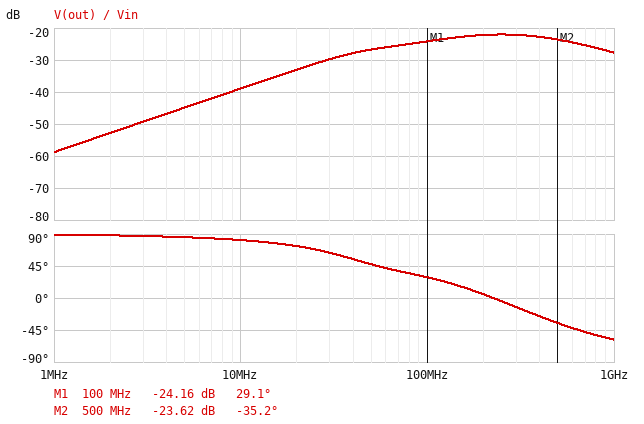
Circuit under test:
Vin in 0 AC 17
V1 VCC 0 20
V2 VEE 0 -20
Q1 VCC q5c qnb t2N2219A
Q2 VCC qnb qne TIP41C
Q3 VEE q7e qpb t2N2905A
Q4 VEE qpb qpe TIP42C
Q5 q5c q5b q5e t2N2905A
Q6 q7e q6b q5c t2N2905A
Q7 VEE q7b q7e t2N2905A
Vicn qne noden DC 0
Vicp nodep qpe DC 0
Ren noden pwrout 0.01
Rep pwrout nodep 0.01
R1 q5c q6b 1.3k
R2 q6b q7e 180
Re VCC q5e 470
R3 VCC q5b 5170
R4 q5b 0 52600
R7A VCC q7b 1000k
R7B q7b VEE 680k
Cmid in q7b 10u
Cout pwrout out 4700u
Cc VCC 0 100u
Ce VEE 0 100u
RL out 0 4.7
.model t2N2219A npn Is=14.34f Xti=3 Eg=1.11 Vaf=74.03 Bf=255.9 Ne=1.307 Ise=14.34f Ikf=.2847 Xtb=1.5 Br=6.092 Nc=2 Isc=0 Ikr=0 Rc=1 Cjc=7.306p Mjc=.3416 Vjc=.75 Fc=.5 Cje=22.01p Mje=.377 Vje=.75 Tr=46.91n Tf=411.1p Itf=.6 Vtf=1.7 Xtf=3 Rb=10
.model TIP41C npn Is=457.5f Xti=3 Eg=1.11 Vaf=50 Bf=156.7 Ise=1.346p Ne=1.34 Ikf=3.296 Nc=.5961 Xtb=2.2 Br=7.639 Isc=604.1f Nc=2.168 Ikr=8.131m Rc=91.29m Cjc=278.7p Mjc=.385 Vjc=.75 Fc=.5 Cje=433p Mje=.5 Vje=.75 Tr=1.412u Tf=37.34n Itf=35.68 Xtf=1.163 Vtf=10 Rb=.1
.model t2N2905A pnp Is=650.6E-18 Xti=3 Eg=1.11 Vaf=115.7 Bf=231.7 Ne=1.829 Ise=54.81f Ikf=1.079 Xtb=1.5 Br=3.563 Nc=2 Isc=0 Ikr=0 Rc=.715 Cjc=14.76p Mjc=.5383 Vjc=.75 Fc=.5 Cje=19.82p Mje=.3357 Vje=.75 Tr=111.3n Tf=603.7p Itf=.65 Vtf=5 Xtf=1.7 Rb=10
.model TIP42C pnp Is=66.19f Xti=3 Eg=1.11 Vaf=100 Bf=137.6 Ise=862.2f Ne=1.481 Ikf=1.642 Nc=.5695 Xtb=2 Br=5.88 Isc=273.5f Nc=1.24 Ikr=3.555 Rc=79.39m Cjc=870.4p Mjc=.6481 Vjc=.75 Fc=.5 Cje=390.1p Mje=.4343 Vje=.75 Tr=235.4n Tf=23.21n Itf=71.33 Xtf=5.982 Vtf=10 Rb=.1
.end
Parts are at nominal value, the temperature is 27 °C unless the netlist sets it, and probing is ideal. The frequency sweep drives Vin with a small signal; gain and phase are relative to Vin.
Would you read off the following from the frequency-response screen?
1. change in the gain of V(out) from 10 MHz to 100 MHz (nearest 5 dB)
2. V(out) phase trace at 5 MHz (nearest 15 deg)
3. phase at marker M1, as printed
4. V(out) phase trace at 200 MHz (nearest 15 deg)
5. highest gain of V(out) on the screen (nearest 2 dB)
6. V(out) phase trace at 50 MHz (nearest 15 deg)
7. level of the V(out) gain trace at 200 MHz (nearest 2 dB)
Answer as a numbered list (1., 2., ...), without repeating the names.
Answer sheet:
1. 15 dB
2. 90 deg
3. 29.1 deg
4. 0 deg
5. -22 dB
6. 45 deg
7. -22 dB
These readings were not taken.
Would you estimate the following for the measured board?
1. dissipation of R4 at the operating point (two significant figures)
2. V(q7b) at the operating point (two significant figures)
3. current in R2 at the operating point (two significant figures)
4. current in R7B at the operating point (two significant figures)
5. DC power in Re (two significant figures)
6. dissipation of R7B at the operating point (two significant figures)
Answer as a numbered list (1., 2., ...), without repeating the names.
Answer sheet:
1. 6.3 mW
2. -480 mV
3. 570 µA
4. 29 µA
5. 2.2 mW
6. 560 µW
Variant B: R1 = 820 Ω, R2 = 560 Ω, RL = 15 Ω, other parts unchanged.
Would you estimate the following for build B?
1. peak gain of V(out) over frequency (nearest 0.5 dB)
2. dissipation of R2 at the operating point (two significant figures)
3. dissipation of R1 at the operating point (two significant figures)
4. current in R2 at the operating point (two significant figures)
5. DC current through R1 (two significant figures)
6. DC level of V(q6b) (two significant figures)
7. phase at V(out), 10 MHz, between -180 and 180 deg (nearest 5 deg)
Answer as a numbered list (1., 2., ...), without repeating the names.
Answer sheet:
1. -18.5 dB
2. 450 µW
3. 650 µW
4. 900 µA
5. 890 µA
6. 760 mV
7. 70 deg
